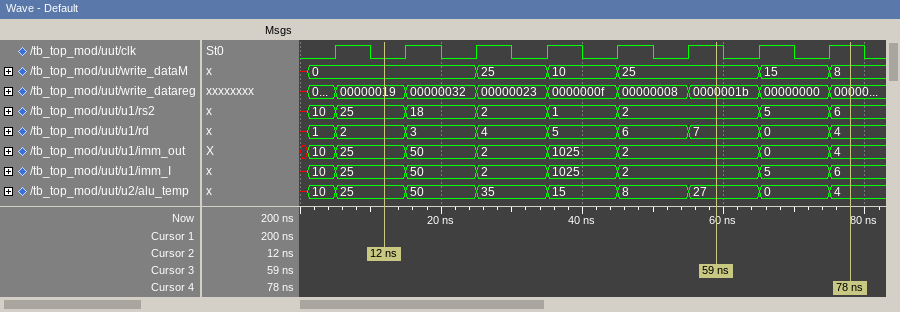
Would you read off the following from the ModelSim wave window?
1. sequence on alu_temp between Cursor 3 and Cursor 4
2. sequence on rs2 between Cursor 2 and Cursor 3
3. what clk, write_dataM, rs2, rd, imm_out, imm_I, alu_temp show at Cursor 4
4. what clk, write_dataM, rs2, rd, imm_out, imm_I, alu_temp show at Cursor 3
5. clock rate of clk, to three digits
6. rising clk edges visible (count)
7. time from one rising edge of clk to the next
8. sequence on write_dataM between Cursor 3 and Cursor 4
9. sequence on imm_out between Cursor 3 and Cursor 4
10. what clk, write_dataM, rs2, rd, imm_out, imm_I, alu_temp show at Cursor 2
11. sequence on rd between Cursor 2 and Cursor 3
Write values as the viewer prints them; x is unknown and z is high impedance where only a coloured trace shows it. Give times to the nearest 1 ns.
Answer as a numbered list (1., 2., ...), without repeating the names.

1. 27, 0, 4
2. 25, 18, 2, 1, 2
3. clk=1, write_dataM=8, rs2=6, rd=4, imm_out=4, imm_I=6, alu_temp=4
4. clk=1, write_dataM=25, rs2=2, rd=7, imm_out=2, imm_I=2, alu_temp=27
5. 100 MHz
6. 8
7. 10 ns
8. 25, 15, 8
9. 2, 0, 4
10. clk=0, write_dataM=0, rs2=25, rd=2, imm_out=25, imm_I=25, alu_temp=25
11. 2, 3, 4, 5, 6, 7
